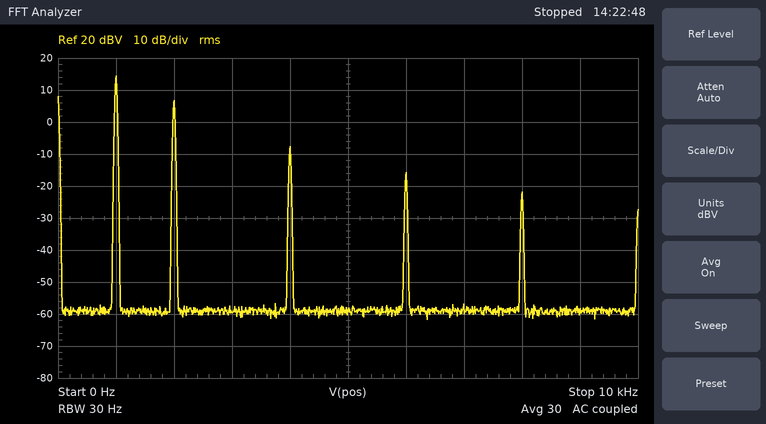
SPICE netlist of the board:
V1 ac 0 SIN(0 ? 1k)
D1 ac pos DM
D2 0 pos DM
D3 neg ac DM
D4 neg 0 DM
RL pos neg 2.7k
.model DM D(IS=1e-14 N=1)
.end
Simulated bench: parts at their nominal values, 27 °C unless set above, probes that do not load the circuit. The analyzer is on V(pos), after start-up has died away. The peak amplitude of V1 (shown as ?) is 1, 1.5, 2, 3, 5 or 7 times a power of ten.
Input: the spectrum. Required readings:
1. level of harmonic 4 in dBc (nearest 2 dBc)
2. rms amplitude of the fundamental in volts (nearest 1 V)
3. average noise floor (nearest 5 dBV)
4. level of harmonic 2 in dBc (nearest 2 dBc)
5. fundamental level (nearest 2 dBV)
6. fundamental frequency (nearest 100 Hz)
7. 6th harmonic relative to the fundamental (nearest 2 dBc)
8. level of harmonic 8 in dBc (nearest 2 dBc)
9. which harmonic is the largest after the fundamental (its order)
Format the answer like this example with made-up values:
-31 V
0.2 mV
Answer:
-22 dBc
5 V
-60 dBV
-8 dBc
14 dBV
1.0 kHz
-30 dBc
-36 dBc
2
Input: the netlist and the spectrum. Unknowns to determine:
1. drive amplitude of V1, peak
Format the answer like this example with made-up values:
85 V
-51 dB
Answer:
15 V
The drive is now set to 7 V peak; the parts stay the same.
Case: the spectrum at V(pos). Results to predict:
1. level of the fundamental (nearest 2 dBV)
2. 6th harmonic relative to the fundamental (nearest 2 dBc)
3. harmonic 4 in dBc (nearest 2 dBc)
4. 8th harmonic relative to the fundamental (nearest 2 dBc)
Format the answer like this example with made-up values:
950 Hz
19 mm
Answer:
8 dBV
-36 dBc
-24 dBc
-50 dBc
